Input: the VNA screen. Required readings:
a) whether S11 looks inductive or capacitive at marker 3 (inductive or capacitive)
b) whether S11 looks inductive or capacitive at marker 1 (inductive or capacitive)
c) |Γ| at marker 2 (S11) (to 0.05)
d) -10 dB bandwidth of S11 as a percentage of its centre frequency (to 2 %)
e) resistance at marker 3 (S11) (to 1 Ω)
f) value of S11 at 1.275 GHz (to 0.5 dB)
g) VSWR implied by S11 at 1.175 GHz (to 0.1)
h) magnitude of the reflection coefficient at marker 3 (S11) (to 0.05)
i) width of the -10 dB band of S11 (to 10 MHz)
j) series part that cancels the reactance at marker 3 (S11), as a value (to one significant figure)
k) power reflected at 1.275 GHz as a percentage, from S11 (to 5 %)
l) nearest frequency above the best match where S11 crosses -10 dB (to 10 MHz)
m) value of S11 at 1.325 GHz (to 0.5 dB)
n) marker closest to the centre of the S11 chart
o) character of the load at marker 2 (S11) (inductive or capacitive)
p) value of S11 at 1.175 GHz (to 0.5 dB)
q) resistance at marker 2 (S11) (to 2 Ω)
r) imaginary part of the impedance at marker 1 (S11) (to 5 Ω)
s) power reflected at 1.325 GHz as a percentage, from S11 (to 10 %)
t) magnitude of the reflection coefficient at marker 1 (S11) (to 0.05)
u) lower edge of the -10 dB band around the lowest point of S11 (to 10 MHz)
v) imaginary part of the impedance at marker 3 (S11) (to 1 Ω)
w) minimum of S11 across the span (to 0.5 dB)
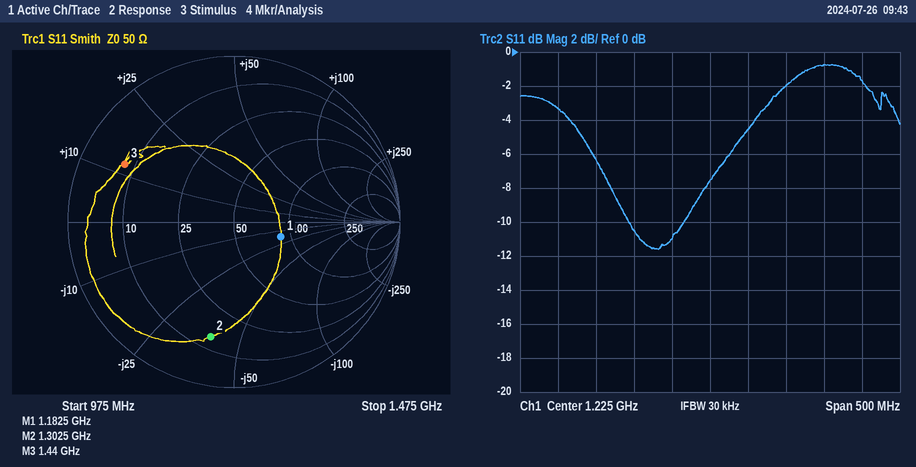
inductive
capacitive
0.70
6 %
8 Ω
-4.5 dB
1.8
0.75
70 MHz
9 pF
35 %
1.19 GHz
-2.0 dB
marker 1
capacitive
-11.0 dB
14 Ω
-15 Ω
60 %
0.30
1.12 GHz
+12 Ω
-11.5 dB
